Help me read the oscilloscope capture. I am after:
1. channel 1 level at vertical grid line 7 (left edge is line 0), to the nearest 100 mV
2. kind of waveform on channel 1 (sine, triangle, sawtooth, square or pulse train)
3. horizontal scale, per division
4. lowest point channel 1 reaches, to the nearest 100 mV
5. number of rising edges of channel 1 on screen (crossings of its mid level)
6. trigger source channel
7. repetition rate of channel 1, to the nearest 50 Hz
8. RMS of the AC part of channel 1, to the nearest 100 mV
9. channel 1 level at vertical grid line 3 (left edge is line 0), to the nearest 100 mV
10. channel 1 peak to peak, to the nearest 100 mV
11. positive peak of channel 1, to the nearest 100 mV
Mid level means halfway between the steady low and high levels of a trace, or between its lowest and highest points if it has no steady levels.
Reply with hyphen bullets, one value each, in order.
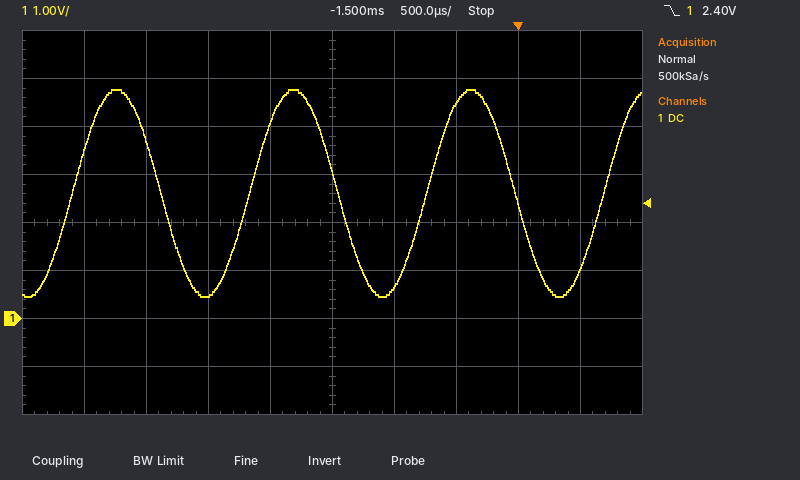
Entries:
- 4.5 V
- sine
- 500 µs
- 500 mV
- 4
- channel 1
- 700 Hz
- 1.5 V
- 500 mV
- 4.3 V
- 4.8 V
